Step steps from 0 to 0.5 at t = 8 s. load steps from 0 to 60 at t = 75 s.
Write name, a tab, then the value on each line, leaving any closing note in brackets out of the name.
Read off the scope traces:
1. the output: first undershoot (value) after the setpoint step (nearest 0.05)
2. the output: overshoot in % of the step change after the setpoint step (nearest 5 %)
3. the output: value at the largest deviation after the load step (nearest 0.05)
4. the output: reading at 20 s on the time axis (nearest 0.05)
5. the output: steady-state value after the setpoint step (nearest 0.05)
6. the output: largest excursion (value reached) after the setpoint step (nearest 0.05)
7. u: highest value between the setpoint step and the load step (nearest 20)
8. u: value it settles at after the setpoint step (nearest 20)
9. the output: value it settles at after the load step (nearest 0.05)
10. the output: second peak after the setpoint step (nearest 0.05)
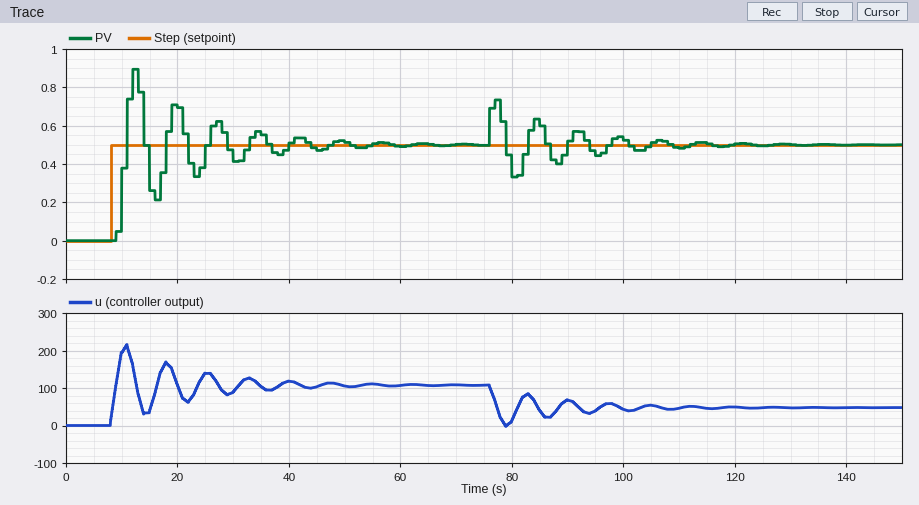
the output: first undershoot (value) after the setpoint step	0.20
the output: overshoot in % of the step change after the setpoint step	80 %
the output: value at the largest deviation after the load step	0.75
the output: reading at 20 s on the time axis	0.70
the output: steady-state value after the setpoint step	0.50
the output: largest excursion (value reached) after the setpoint step	0.90
u: highest value between the setpoint step and the load step	220
u: value it settles at after the setpoint step	100
the output: value it settles at after the load step	0.50
the output: second peak after the setpoint step	0.70
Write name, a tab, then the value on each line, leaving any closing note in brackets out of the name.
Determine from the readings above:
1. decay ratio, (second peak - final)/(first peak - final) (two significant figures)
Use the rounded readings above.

decay ratio, (second peak - final)/(first peak - final)	0.50
